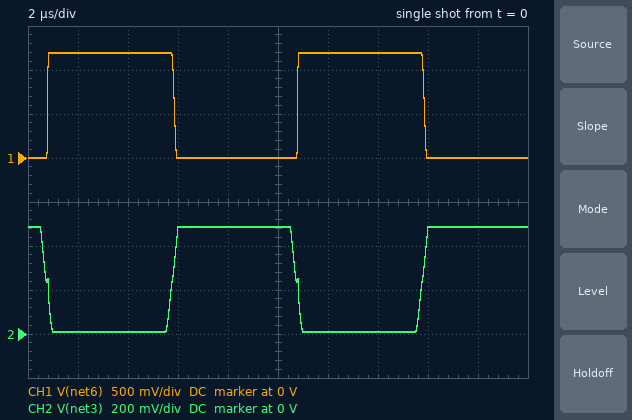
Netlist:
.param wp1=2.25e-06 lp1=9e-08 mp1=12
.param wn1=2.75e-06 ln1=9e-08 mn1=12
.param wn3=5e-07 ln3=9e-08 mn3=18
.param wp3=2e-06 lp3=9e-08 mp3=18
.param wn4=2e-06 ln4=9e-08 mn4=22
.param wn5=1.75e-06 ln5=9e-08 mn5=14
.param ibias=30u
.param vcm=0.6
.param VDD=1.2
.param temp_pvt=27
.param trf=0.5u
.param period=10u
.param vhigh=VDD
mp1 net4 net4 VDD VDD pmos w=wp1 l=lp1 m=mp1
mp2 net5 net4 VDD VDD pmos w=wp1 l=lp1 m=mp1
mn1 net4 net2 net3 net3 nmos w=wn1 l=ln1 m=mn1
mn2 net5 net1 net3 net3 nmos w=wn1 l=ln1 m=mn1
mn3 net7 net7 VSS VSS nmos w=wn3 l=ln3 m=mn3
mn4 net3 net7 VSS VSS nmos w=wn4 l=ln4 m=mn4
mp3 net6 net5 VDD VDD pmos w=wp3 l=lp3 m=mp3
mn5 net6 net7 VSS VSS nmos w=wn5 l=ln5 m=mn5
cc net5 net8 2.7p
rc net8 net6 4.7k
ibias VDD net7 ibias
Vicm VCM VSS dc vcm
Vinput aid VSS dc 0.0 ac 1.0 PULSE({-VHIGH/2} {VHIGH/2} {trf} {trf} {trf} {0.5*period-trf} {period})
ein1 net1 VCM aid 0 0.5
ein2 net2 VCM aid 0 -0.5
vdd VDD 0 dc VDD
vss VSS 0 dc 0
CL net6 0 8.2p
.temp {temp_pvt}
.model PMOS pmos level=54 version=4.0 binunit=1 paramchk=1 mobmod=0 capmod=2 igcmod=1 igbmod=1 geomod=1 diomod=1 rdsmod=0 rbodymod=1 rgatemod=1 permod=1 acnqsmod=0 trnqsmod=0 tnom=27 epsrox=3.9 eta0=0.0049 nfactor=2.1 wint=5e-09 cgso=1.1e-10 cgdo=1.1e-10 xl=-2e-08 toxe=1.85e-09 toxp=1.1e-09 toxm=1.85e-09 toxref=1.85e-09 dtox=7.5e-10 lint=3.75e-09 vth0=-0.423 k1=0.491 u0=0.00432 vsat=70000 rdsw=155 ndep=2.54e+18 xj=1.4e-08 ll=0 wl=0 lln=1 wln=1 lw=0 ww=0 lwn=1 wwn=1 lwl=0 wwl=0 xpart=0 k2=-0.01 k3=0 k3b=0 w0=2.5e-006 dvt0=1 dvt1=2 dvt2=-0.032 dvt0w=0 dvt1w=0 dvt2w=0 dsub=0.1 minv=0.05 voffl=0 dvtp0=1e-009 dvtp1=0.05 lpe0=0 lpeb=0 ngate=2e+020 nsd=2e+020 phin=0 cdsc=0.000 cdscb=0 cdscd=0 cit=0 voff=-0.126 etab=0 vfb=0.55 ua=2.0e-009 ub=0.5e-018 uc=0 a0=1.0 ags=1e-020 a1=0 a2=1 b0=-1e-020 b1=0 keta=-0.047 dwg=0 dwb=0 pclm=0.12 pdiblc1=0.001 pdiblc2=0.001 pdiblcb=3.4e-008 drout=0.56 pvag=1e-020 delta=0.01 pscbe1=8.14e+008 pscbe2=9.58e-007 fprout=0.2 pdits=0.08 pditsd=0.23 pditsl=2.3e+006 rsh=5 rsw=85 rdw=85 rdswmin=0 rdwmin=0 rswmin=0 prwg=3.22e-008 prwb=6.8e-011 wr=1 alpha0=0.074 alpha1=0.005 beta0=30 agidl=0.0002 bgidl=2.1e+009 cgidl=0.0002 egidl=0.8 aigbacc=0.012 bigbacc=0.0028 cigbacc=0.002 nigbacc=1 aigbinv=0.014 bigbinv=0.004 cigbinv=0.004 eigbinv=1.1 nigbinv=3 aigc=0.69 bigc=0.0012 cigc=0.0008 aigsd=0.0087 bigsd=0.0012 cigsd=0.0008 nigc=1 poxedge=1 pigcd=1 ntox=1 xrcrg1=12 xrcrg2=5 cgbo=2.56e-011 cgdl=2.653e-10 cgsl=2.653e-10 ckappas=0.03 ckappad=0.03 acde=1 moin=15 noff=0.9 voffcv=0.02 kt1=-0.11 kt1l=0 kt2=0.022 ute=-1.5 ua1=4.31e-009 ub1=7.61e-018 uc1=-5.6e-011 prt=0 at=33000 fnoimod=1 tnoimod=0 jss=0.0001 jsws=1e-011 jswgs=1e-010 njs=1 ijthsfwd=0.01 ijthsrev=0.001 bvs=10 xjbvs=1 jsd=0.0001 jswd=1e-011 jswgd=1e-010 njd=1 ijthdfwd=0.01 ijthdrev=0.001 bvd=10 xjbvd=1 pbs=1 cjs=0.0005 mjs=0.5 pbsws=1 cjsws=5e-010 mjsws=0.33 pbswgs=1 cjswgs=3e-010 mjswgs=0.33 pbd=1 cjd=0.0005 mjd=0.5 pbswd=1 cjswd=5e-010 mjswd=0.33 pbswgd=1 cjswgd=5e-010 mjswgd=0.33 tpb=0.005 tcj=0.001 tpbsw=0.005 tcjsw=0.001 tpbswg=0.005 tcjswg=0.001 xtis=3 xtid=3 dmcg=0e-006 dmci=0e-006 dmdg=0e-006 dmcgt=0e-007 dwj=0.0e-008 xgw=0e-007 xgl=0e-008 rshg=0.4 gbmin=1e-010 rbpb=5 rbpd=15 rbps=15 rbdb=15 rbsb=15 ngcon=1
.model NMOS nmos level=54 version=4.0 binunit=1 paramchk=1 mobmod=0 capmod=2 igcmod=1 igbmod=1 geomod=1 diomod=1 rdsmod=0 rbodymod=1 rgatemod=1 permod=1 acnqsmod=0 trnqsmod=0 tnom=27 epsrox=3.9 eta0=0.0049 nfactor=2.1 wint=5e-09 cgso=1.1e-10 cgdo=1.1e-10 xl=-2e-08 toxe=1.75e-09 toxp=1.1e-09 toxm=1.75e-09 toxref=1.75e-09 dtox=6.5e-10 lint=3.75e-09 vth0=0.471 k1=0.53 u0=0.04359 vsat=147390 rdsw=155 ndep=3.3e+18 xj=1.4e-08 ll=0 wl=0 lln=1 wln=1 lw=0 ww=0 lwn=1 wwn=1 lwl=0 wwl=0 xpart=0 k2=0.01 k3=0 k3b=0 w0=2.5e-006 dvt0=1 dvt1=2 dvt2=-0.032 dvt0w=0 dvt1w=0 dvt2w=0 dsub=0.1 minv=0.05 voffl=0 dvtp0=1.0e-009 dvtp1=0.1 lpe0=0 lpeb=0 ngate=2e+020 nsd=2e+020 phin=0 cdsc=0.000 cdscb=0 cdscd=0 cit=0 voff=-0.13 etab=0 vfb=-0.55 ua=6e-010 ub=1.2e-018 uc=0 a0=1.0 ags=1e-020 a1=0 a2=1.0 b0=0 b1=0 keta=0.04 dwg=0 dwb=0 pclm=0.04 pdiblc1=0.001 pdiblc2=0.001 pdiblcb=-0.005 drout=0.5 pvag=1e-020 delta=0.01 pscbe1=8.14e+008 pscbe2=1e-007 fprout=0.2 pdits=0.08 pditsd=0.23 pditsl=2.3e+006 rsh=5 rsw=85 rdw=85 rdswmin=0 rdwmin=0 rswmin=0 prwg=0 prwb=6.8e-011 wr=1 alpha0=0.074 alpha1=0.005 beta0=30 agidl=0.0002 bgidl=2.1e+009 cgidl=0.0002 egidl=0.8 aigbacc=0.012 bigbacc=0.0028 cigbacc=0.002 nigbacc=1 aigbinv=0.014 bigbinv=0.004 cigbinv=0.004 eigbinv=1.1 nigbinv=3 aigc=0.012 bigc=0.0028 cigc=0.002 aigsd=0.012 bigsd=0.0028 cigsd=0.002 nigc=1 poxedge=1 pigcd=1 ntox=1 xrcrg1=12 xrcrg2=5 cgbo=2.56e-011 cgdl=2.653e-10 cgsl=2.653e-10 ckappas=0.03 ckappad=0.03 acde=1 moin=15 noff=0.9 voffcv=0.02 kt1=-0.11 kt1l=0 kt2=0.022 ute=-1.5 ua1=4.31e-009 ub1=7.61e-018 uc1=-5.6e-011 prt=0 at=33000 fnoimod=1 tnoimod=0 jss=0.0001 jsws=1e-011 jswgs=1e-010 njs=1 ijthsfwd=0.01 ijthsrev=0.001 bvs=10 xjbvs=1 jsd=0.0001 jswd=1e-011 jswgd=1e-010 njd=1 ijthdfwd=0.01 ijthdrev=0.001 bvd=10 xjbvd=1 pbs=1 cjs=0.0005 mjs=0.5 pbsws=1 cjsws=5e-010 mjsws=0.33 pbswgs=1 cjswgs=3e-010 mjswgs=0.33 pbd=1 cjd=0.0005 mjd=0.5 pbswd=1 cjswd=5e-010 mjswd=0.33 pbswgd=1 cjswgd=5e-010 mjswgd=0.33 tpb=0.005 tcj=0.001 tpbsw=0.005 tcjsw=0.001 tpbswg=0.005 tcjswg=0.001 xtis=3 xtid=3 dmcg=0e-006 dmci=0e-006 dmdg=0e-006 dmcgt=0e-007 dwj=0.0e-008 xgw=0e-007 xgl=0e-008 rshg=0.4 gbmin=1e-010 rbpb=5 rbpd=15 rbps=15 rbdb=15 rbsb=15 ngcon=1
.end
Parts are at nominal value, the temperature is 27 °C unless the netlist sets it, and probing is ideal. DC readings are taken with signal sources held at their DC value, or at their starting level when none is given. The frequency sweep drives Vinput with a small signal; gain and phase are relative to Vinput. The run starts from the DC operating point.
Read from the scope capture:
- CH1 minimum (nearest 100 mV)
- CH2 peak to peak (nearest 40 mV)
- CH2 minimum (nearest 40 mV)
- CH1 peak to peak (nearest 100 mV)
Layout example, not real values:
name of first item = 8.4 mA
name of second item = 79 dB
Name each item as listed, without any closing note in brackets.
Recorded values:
CH1 minimum = 0 V
CH2 peak to peak = 480 mV
CH2 minimum = 0 V
CH1 peak to peak = 1.2 V
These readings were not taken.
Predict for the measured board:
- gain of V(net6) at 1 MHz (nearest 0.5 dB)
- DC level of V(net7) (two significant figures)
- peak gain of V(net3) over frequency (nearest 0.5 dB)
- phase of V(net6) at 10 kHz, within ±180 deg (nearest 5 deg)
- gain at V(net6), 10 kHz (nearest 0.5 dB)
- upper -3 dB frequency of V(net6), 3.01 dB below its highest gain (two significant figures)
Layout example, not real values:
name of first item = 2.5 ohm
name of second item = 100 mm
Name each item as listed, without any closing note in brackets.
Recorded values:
gain of V(net6) at 1 MHz = 37.0 dB
DC level of V(net7) = 390 mV
peak gain of V(net3) over frequency = -12.0 dB
phase of V(net6) at 10 kHz, within ±180 deg = -5 deg
gain at V(net6), 10 kHz = 57.0 dB
upper -3 dB frequency of V(net6), 3.01 dB below its highest gain = 98 kHz
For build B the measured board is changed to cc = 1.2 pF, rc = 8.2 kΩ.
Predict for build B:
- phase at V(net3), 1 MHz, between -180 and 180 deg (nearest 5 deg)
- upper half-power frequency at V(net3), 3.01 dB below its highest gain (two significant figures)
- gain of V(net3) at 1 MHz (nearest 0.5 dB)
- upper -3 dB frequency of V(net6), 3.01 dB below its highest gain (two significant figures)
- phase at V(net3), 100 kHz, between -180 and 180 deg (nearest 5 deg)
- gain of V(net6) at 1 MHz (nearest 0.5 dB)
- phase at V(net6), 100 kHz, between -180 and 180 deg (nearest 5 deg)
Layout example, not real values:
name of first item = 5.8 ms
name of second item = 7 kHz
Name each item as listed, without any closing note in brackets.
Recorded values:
phase at V(net3), 1 MHz, between -180 and 180 deg = 150 deg
upper half-power frequency at V(net3), 3.01 dB below its highest gain = 210 kHz
gain of V(net3) at 1 MHz = -23.0 dB
upper -3 dB frequency of V(net6), 3.01 dB below its highest gain = 200 kHz
phase at V(net3), 100 kHz, between -180 and 180 deg = 160 deg
gain of V(net6) at 1 MHz = 43.0 dB
phase at V(net6), 100 kHz, between -180 and 180 deg = -25 deg
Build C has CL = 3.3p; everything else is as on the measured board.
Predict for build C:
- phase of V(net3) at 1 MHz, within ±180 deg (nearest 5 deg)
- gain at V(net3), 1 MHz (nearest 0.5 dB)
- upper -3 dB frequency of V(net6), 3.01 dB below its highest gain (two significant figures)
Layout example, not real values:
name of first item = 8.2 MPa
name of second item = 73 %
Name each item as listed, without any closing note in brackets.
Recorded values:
phase of V(net3) at 1 MHz, within ±180 deg = 130 deg
gain at V(net3), 1 MHz = -30.5 dB
upper -3 dB frequency of V(net6), 3.01 dB below its highest gain = 100 kHz
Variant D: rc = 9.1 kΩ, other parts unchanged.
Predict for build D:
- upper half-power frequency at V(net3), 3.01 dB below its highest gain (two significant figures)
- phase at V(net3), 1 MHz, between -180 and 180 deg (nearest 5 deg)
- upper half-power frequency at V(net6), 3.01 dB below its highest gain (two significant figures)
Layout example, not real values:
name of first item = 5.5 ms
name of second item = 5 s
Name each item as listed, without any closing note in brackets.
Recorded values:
upper half-power frequency at V(net3), 3.01 dB below its highest gain = 98 kHz
phase at V(net3), 1 MHz, between -180 and 180 deg = 150 deg
upper half-power frequency at V(net6), 3.01 dB below its highest gain = 97 kHz
